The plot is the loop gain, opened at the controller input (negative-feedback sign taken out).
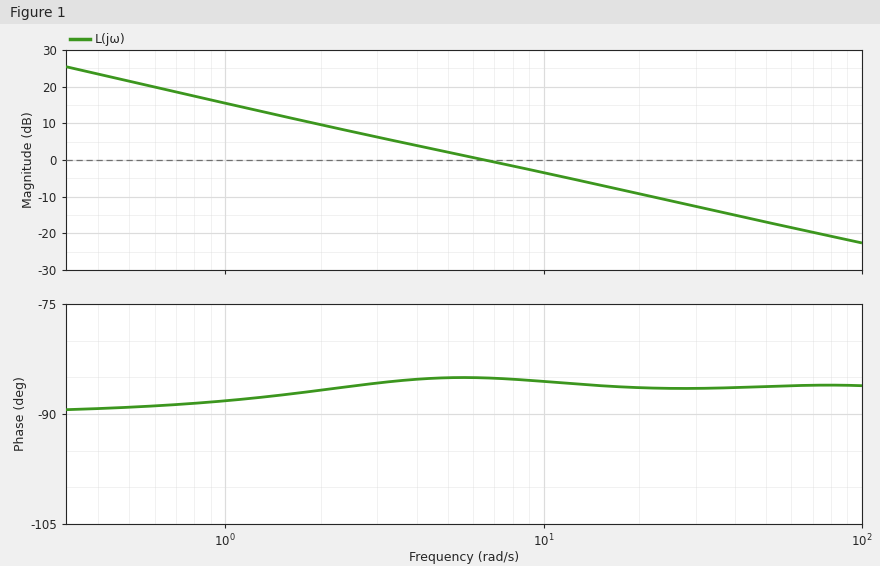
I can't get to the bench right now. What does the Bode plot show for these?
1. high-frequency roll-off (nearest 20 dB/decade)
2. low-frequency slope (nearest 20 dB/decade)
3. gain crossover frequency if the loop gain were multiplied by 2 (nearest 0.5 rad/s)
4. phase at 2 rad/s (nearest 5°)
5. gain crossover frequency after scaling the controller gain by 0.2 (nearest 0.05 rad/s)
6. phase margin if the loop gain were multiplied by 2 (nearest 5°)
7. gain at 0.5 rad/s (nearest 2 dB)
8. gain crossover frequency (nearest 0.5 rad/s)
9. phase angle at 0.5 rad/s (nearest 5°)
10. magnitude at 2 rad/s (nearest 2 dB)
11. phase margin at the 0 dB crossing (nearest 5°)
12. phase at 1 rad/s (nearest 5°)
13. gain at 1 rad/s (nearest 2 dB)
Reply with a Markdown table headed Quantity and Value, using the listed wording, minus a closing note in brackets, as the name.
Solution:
| Quantity | Value |
|---|---|
| high-frequency roll-off | -20 dB/decade |
| low-frequency slope | -20 dB/decade |
| gain crossover frequency if the loop gain were multiplied by 2 | 13.5 rad/s |
| phase at 2 rad/s | -85° |
| gain crossover frequency after scaling the controller gain by 0.2 | 1.20 rad/s |
| phase margin if the loop gain were multiplied by 2 | 95° |
| gain at 0.5 rad/s | 22 dB |
| gain crossover frequency | 6.5 rad/s |
| phase angle at 0.5 rad/s | -90° |
| magnitude at 2 rad/s | 10 dB |
| phase margin at the 0 dB crossing | 95° |
| phase at 1 rad/s | -90° |
| gain at 1 rad/s | 16 dB |
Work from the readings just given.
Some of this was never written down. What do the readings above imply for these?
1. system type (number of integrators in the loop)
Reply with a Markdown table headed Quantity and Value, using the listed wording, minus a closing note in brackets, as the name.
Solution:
| Quantity | Value |
|---|---|
| system type | 1 |
